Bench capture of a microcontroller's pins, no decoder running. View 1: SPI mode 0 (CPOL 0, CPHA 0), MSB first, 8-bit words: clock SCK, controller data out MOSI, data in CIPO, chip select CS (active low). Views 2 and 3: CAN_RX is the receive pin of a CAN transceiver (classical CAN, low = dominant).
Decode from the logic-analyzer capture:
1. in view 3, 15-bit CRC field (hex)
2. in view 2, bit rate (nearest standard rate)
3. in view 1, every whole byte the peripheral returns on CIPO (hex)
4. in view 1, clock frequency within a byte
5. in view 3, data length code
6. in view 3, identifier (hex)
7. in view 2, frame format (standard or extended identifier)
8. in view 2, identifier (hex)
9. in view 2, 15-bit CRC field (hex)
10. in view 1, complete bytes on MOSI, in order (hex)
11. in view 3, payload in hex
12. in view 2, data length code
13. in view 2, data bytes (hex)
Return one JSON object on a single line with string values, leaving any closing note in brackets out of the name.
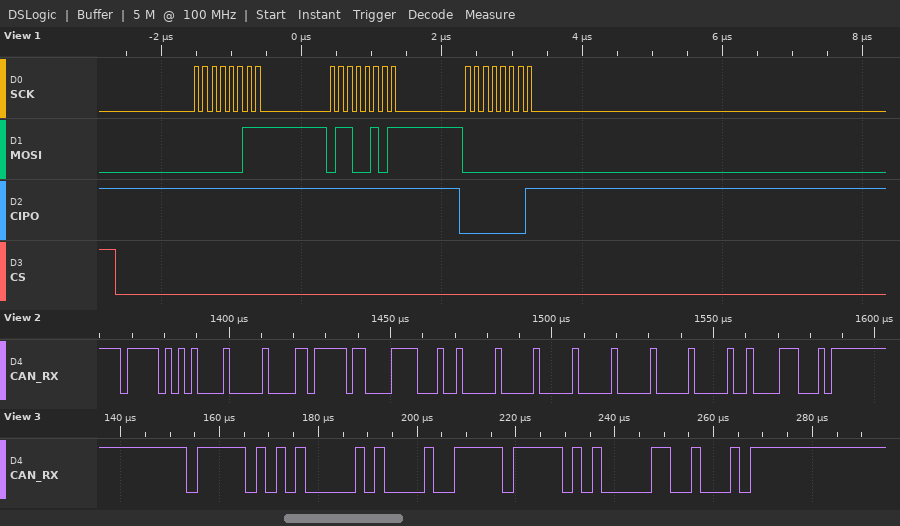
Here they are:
{"in view 3, 15-bit CRC field": "0x5048", "in view 2, bit rate": "500 kbit/s", "in view 1, every whole byte the peripheral returns on CIPO": "FF FF 01", "in view 1, clock frequency within a byte": "8 MHz", "in view 3, data length code": "2", "in view 3, identifier": "0x7EA", "in view 2, frame format": "standard", "in view 2, identifier": "0x7EA", "in view 2, 15-bit CRC field": "0x0438", "in view 1, complete bytes on MOSI, in order": "03 65 00", "in view 3, payload in hex": "13 FF", "in view 2, data length code": "8", "in view 2, data bytes": "03 7F 0F 12 00 00 00 00"}
